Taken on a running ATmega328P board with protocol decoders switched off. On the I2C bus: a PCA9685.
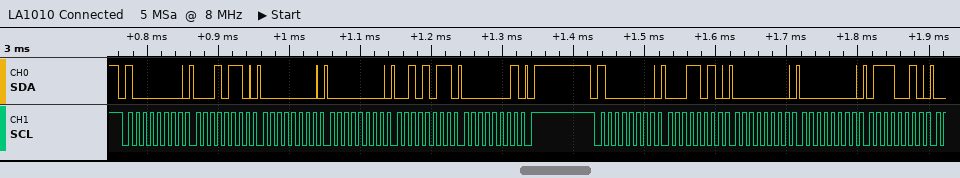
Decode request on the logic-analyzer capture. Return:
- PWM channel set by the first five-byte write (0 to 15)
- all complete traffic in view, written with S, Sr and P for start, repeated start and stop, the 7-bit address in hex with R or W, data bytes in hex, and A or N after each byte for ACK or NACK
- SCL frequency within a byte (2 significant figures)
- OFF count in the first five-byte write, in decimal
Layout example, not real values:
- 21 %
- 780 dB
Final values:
- 4
- S 40W A 16 A 00 A 00 A 2B A 01 A P S 40W A 1A A 00 A 00 A 72 A
- 100 kHz
- 299
